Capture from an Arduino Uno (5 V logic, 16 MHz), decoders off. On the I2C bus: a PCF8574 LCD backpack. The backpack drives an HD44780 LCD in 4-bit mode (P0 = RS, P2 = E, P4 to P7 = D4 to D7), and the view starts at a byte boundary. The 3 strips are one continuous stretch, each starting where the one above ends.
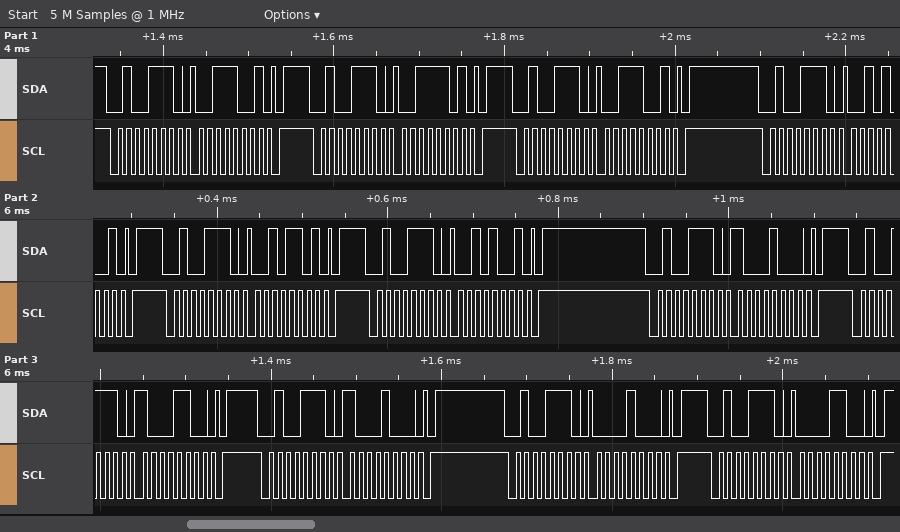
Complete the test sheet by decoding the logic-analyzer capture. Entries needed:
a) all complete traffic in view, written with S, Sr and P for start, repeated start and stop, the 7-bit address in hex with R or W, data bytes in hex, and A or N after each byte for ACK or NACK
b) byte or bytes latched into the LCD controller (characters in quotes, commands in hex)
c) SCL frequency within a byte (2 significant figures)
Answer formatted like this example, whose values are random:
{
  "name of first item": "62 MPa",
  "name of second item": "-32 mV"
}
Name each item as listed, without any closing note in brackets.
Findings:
{
  "all complete traffic in view, written with S, Sr and P for start, repeated start and stop, the 7-bit address in hex with R or W, data bytes in hex, and A or N after each byte for ACK or NACK": "S 27W A 39 A P S 27W A 3D A P S 27W A 39 A P S 27W A 29 A P S 27W A 2D A P S 27W A 29 A P S 27W A 88 A P S 27W A 8C A P S 27W A 88 A P S 27W A 08 A P S 27W A 0C A P",
  "byte or bytes latched into the LCD controller": "'2'",
  "SCL frequency within a byte": "100 kHz"
}
